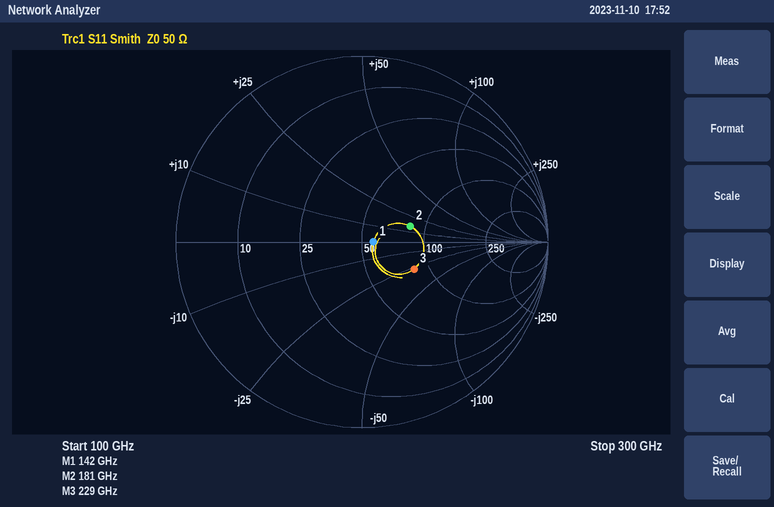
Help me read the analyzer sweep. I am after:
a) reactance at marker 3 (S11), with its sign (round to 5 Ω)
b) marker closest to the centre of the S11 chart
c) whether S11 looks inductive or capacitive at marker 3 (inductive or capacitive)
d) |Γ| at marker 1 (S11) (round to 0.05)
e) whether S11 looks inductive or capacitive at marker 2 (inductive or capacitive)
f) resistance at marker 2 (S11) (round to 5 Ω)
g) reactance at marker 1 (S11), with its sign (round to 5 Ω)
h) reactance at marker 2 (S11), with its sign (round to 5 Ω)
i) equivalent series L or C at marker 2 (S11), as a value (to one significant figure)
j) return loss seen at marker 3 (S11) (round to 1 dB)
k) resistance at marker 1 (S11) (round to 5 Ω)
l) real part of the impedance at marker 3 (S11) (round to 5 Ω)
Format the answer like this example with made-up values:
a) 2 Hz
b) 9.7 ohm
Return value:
a) -25 Ω
b) marker 1
c) capacitive
d) 0.05
e) inductive
f) 85 Ω
g) 0 Ω
h) +15 Ω
i) 10 pH
j) 10 dB
k) 55 Ω
l) 85 Ω
